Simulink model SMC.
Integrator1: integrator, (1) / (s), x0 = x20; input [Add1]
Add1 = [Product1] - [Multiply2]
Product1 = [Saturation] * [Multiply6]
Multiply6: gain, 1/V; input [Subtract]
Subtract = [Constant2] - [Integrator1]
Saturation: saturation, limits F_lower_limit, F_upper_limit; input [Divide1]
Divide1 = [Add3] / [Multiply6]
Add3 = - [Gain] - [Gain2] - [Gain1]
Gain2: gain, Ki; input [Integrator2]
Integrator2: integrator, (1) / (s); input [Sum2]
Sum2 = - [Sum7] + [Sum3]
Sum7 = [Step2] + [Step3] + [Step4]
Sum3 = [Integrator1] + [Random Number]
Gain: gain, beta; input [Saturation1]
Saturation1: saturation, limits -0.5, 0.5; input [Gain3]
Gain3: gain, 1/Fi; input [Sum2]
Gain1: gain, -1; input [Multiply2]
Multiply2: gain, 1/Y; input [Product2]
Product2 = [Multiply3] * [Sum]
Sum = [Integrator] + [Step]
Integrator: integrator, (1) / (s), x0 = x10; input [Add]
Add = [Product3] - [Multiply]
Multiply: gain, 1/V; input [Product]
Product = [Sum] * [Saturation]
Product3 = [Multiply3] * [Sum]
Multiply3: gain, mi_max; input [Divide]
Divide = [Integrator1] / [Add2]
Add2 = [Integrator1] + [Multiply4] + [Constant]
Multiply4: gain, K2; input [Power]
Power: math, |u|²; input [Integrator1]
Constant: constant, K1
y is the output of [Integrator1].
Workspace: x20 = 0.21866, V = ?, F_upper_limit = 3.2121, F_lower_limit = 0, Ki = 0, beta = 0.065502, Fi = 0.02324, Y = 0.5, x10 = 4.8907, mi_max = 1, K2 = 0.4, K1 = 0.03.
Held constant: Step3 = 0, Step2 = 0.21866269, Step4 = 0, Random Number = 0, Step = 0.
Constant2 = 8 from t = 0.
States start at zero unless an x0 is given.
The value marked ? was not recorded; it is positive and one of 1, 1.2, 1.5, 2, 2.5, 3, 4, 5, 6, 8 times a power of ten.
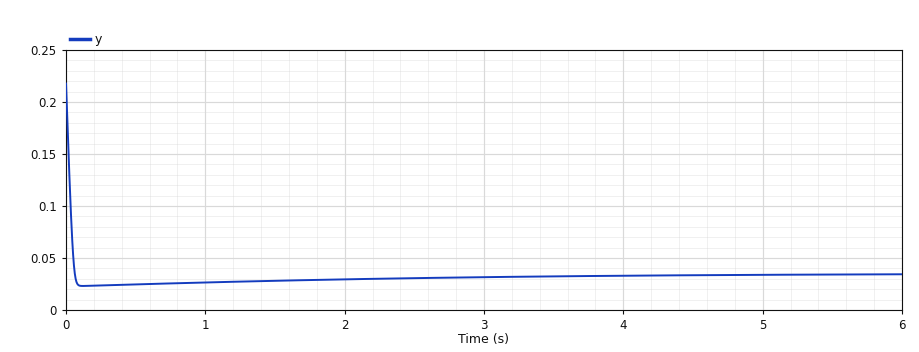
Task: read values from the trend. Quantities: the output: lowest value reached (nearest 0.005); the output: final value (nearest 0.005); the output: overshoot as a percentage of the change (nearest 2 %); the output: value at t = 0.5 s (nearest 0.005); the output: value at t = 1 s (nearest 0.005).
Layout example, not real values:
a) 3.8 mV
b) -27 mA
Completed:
a) 0.025
b) 0.035
c) 6 %
d) 0.025
e) 0.025
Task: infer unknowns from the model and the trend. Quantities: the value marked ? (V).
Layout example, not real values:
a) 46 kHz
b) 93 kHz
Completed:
a) 6
